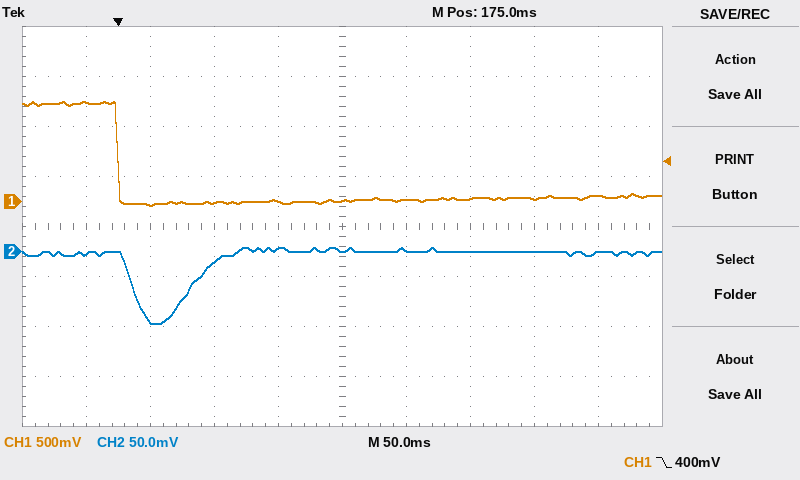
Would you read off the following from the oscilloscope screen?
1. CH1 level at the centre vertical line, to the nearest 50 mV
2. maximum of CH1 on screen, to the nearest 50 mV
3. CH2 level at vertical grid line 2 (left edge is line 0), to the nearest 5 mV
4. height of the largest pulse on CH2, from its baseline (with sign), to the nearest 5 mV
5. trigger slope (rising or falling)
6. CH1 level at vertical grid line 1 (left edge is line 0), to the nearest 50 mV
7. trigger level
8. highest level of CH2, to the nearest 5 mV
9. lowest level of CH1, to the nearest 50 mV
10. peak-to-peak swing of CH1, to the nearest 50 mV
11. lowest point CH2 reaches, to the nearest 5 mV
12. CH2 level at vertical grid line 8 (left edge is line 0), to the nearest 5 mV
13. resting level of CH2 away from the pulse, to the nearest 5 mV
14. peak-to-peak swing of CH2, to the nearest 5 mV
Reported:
0 mV
1.00 V
-70 mV
-70 mV
falling
1.00 V
400 mV
5 mV
-50 mV
1.05 V
-70 mV
0 mV
0 mV
75 mV
